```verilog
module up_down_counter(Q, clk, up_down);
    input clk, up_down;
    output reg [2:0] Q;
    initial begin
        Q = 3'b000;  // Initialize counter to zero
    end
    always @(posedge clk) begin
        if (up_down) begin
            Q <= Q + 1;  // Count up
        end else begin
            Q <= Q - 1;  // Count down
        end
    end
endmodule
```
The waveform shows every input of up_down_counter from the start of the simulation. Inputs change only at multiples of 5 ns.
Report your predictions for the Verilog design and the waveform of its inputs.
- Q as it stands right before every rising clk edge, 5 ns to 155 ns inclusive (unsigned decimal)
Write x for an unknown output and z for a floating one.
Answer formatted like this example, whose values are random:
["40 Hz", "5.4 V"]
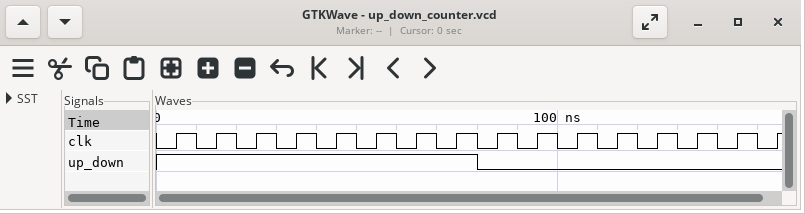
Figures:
["0, 1, 2, 3, 4, 5, 6, 7, 0, 7, 6, 5, 4, 3, 2, 1"]
